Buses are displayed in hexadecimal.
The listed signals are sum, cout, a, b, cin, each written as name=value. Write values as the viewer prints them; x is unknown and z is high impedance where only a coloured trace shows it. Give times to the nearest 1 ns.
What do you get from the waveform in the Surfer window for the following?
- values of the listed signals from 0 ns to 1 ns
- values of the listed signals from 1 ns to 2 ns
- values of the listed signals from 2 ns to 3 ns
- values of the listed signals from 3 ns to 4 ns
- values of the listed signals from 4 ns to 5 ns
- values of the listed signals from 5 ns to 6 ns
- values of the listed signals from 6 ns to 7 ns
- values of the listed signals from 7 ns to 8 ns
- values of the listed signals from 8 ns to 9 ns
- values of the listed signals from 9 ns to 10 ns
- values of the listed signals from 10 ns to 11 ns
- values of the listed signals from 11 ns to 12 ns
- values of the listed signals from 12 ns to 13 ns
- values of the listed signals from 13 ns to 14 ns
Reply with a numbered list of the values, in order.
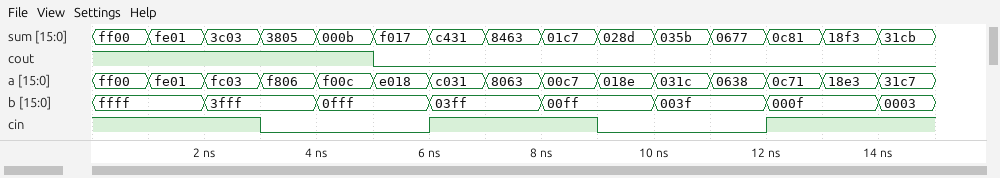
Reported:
1. sum=ff00, cout=1, a=ff00, b=ffff, cin=1
2. sum=fe01, cout=1, a=fe01, b=ffff, cin=1
3. sum=3c03, cout=1, a=fc03, b=3fff, cin=1
4. sum=3805, cout=1, a=f806, b=3fff, cin=0
5. sum=000b, cout=1, a=f00c, b=0fff, cin=0
6. sum=f017, cout=0, a=e018, b=0fff, cin=0
7. sum=c431, cout=0, a=c031, b=03ff, cin=1
8. sum=8463, cout=0, a=8063, b=03ff, cin=1
9. sum=01c7, cout=0, a=00c7, b=00ff, cin=1
10. sum=028d, cout=0, a=018e, b=00ff, cin=0
11. sum=035b, cout=0, a=031c, b=003f, cin=0
12. sum=0677, cout=0, a=0638, b=003f, cin=0
13. sum=0c81, cout=0, a=0c71, b=000f, cin=1
14. sum=18f3, cout=0, a=18e3, b=000f, cin=1
